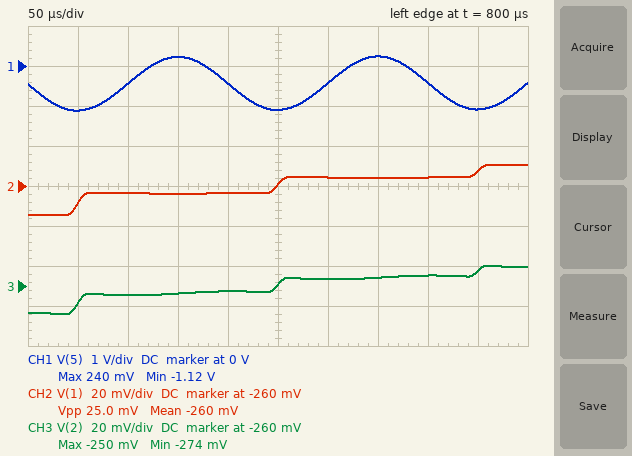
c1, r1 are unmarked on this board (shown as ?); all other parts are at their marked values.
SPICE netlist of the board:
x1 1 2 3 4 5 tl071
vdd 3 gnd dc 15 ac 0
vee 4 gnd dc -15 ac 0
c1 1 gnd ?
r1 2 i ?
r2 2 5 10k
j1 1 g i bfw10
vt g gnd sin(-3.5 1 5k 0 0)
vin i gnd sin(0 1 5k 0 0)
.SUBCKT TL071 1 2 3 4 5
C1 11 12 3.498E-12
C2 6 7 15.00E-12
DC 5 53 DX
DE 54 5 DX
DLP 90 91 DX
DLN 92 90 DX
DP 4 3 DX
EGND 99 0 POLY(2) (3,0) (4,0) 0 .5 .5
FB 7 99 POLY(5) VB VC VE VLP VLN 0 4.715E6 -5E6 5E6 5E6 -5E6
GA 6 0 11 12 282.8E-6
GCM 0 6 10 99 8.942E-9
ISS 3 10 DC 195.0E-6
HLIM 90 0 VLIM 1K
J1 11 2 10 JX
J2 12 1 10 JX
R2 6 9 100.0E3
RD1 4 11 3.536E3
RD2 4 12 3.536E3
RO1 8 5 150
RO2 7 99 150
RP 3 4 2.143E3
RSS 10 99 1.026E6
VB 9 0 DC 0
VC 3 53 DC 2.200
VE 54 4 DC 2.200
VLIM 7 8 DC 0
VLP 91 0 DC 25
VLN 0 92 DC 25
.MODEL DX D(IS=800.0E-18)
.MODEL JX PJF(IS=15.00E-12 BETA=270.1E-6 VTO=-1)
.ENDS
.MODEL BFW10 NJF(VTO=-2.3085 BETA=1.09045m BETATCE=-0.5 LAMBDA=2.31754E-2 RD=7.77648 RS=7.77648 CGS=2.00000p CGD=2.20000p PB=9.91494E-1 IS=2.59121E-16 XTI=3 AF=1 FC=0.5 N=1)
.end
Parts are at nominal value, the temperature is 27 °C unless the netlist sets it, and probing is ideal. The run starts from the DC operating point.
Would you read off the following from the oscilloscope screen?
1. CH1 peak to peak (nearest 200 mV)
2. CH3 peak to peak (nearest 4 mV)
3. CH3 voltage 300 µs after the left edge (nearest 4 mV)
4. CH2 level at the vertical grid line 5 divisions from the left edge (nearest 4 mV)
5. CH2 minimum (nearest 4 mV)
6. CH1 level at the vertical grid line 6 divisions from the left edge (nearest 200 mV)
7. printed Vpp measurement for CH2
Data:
1.4 V
24 mV
-256 mV
-260 mV
-276 mV
-400 mV
25.0 mV
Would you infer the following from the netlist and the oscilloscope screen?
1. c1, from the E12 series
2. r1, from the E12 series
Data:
8.2 nF
15 kΩ
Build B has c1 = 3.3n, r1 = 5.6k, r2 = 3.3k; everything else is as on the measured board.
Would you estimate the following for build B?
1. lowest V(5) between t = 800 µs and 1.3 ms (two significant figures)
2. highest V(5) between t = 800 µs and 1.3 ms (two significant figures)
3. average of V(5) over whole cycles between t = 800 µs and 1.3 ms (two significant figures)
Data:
-960 mV
230 mV
-370 mV
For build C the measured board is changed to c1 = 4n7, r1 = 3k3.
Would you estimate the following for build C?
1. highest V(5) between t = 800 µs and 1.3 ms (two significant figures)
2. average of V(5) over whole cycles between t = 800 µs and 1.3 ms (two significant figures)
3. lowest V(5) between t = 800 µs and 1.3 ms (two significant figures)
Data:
2.1 V
-970 mV
-4.0 V
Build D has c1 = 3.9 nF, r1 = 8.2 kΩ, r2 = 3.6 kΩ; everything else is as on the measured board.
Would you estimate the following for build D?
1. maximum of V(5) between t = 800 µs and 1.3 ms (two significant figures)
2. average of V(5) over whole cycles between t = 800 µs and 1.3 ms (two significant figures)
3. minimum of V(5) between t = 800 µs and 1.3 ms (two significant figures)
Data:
110 mV
-340 mV
-780 mV
